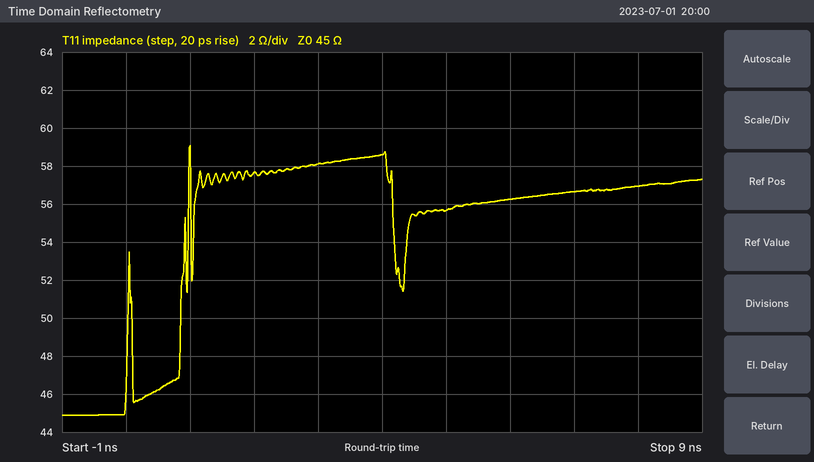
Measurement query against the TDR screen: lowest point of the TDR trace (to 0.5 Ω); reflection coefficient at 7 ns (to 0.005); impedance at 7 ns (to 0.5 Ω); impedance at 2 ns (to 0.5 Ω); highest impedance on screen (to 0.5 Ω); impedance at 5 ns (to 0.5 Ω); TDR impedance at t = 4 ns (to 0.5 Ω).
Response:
45.0 Ω
+0.115
56.5 Ω
57.5 Ω
59.0 Ω
55.5 Ω
58.5 Ω
